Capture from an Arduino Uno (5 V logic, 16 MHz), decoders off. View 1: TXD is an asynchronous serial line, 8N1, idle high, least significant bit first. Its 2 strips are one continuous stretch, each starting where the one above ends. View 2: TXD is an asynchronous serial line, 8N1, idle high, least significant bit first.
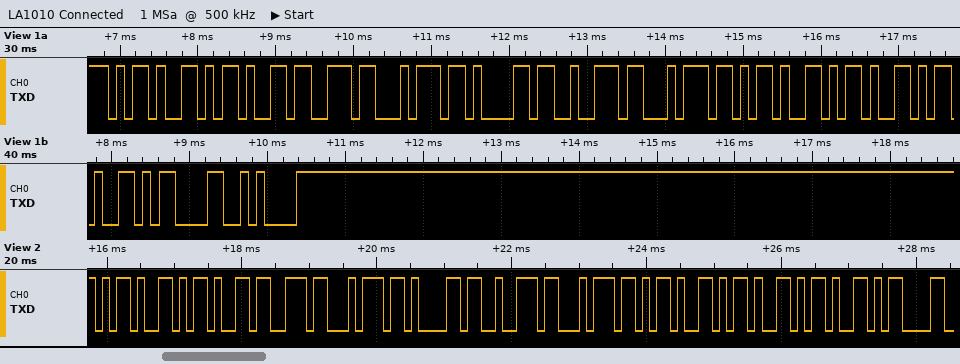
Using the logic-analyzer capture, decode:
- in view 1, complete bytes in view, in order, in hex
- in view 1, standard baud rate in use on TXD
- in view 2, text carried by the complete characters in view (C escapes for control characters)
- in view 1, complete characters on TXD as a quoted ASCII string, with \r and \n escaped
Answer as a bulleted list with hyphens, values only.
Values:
- 0x2D 0x2D 0x73 0x74 0x61 0x72 0x74 0x2D 0x2D 0x2D 0x0D 0x0A
- 9600 baud
- "--start---\r"
- "--start---\r\n"
